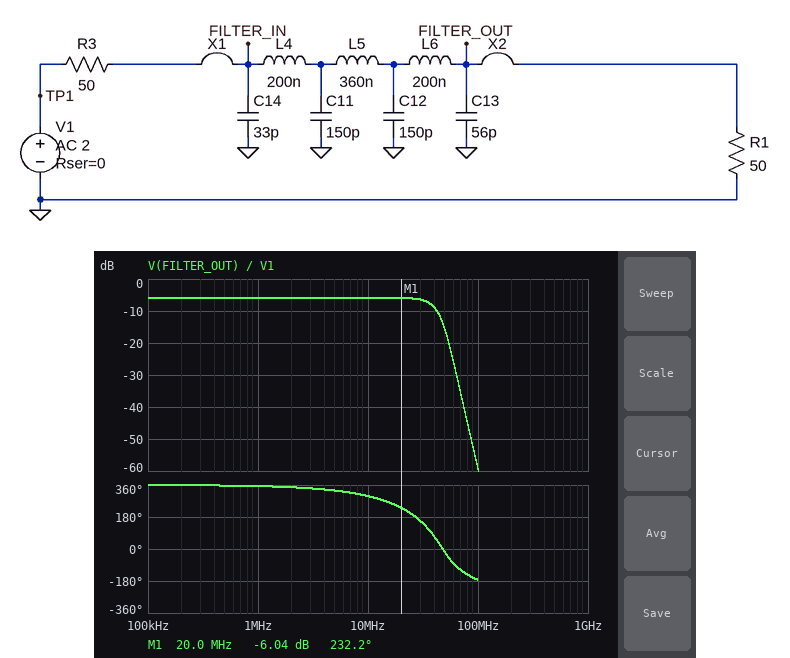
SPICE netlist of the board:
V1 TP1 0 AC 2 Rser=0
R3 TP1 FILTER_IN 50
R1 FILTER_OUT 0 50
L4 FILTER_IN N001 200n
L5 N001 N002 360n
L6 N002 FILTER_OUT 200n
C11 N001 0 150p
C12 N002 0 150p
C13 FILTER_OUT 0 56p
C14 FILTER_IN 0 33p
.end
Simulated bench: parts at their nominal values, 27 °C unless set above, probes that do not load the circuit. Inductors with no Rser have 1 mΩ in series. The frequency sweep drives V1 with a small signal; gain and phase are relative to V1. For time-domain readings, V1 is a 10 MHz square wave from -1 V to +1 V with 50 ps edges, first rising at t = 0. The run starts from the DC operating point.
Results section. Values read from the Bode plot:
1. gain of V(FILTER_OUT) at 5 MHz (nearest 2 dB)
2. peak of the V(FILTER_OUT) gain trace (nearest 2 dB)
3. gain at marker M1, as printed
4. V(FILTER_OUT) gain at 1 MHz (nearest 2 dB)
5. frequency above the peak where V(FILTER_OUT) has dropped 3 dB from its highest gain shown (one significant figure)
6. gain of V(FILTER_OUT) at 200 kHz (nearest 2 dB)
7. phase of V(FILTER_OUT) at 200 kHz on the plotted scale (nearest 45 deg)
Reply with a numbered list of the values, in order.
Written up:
1. -6 dB
2. -6 dB
3. -6.04 dB
4. -6 dB
5. 40 MHz
6. -6 dB
7. 360 deg
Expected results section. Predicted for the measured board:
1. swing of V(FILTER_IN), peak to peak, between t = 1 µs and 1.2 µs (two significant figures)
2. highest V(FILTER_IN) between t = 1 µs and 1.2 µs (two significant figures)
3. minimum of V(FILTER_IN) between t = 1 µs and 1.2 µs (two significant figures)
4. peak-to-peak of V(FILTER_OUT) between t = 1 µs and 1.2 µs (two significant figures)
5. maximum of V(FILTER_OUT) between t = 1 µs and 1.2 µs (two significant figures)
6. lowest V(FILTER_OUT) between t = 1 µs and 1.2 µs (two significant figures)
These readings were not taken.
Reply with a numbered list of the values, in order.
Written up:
1. 1.7 V
2. 850 mV
3. -850 mV
4. 1.3 V
5. 640 mV
6. -640 mV
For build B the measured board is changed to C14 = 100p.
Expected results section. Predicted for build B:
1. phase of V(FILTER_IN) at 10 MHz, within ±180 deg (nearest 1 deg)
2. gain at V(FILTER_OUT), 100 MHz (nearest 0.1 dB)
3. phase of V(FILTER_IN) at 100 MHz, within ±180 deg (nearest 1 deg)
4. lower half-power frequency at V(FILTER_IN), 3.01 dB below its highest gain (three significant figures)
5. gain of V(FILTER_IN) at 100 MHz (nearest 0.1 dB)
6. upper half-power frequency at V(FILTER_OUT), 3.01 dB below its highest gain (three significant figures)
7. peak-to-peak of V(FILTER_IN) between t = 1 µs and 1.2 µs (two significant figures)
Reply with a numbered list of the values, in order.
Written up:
1. -7 deg
2. -67.2 dB
3. -70 deg
4. 45.0 MHz
5. -9.2 dB
6. 45.9 MHz
7. 1.3 V
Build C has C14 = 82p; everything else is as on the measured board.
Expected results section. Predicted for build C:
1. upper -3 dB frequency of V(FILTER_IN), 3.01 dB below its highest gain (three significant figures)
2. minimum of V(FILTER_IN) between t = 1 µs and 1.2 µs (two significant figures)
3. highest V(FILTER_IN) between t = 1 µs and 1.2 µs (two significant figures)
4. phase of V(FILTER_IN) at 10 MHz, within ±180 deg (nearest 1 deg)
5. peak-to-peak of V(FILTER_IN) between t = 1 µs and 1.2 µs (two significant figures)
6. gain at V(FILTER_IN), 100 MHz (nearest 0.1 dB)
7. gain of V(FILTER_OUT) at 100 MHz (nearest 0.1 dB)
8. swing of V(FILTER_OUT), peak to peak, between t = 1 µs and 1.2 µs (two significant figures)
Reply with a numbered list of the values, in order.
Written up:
1. 69.0 MHz
2. -660 mV
3. 660 mV
4. -5 deg
5. 1.3 V
6. -7.5 dB
7. -65.4 dB
8. 1.3 V
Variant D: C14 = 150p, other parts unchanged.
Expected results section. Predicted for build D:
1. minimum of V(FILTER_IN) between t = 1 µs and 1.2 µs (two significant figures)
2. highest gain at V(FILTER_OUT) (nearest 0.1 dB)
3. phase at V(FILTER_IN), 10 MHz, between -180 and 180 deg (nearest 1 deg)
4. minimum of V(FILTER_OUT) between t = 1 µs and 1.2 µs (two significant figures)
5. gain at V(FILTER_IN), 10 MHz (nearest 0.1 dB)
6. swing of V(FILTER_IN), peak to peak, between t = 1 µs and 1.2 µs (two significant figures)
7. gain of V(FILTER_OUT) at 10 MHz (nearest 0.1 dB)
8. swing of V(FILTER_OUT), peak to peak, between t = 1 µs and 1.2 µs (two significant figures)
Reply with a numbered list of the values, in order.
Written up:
1. -560 mV
2. -6.0 dB
3. -11 deg
4. -610 mV
5. -7.1 dB
6. 1.1 V
7. -6.2 dB
8. 1.2 V
